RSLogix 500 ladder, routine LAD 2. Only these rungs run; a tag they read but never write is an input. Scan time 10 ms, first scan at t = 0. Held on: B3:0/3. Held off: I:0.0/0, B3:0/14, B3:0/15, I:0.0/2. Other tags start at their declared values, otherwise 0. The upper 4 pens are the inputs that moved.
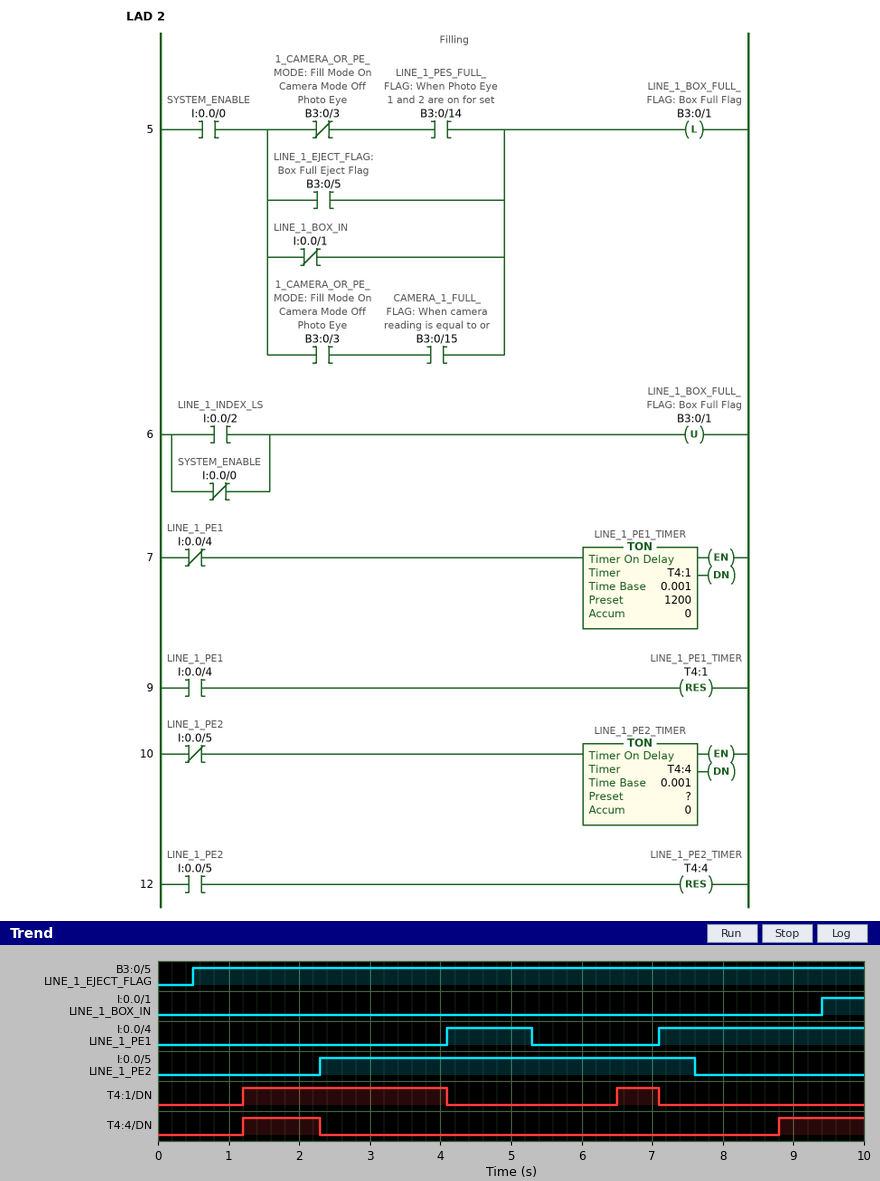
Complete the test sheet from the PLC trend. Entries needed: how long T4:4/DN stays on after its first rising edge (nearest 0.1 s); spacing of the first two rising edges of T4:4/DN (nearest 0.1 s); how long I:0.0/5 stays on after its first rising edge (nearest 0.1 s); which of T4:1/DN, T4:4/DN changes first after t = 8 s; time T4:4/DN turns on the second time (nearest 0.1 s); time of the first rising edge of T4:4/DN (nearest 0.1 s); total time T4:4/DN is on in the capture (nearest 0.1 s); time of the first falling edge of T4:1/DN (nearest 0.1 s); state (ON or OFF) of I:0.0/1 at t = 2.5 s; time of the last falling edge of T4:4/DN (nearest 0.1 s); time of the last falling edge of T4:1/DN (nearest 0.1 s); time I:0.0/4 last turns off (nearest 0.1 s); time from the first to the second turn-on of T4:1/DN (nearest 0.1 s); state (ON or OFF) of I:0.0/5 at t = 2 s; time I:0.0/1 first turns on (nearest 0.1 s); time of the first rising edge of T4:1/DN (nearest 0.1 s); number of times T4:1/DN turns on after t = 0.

1.1 s
7.6 s
5.3 s
T4:4/DN
8.8 s
1.2 s
2.3 s
4.1 s
OFF
2.3 s
7.1 s
5.3 s
5.3 s
OFF
9.4 s
1.2 s
2
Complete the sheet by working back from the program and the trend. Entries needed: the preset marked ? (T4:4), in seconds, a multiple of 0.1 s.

1.2 s
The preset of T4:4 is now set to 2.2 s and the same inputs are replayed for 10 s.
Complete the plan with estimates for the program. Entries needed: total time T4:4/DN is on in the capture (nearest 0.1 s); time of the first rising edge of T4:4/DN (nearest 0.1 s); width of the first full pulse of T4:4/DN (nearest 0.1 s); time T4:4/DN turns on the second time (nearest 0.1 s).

0.3 s
2.2 s
0.1 s
9.8 s
